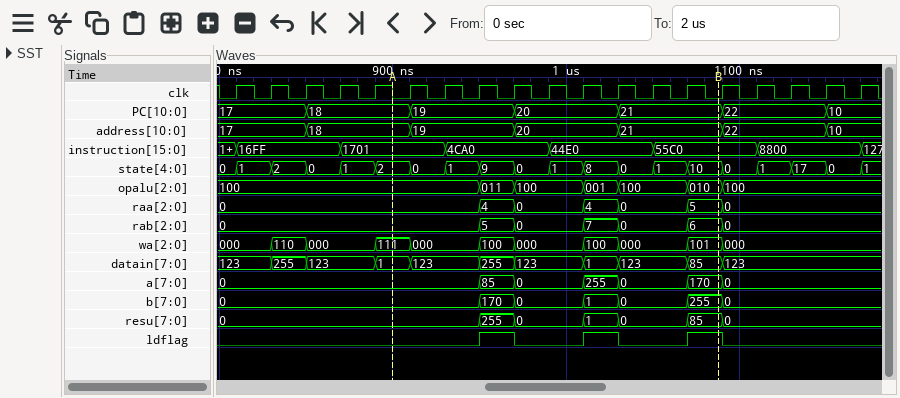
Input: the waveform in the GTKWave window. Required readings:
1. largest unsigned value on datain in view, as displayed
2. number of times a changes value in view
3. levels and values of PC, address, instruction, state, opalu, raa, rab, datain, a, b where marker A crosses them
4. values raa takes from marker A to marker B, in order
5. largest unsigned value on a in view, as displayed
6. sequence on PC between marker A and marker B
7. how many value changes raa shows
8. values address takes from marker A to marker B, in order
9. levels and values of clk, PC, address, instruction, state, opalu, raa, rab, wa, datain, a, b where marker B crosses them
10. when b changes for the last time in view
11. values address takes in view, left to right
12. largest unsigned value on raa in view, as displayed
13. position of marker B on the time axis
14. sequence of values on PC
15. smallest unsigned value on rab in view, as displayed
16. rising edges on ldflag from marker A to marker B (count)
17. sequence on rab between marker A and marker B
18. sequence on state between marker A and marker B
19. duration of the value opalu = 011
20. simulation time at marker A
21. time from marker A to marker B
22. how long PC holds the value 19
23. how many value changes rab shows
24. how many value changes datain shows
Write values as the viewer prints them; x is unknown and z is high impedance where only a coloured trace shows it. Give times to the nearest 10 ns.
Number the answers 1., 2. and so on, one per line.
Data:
1. 255
2. 6
3. PC=18, address=18, instruction=1701, state=2, opalu=100, raa=0, rab=0, datain=1, a=0, b=0
4. 0, 4, 0, 4, 0, 5
5. 255
6. 18, 19, 20, 21
7. 6
8. 18, 19, 20, 21
9. clk=0, PC=21, address=21, instruction=55C0, state=10, opalu=010, raa=5, rab=6, wa=101, datain=85, a=170, b=255
10. 1090 ns
11. 17, 18, 19, 20, 21, 22, 10
12. 5
13. 1090 ns
14. 17, 18, 19, 20, 21, 22, 10
15. 0
16. 3
17. 0, 5, 0, 7, 0, 6
18. 2, 0, 1, 9, 0, 1, 8, 0, 1, 10
19. 20 ns
20. 900 ns
21. 190 ns
22. 60 ns
23. 6
24. 10
